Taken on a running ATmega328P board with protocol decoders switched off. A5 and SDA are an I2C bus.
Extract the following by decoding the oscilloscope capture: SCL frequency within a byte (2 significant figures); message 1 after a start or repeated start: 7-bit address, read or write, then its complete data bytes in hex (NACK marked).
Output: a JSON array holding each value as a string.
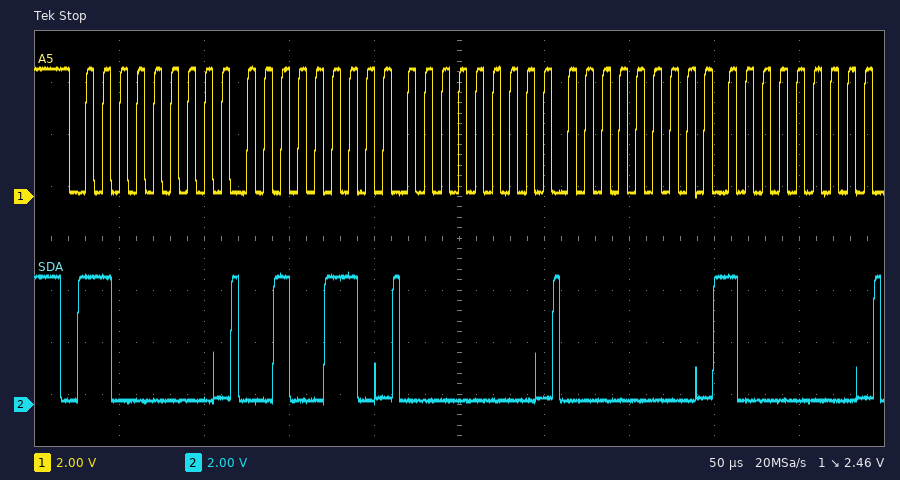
["100 kHz", "0x60 write: 26 00 00 80"]
